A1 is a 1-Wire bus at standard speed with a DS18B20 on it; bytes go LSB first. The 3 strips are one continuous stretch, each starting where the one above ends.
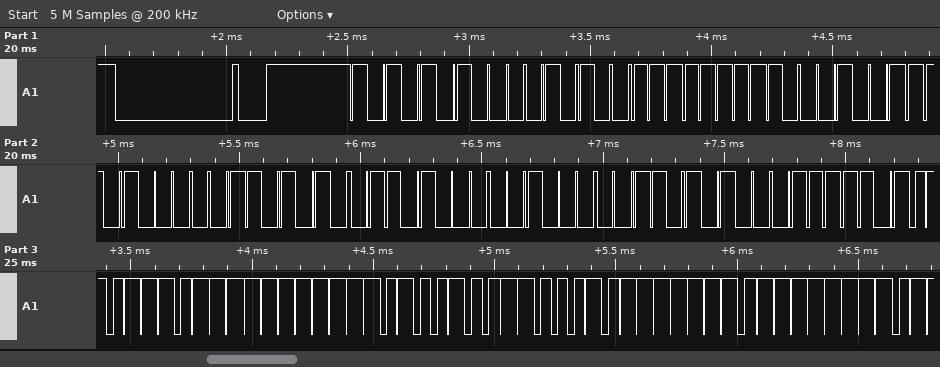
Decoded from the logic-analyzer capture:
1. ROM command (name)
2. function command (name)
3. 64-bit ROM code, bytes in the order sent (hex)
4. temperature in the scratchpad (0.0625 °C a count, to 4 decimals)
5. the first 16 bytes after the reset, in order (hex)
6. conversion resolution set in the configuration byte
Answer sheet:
Match ROM
Read Scratchpad
28 FF 91 0B 56 16 04 2B
-4.3750 °C
55 28 FF 91 0B 56 16 04 2B BE BA FF 4B 46 7F FF
12 bits
